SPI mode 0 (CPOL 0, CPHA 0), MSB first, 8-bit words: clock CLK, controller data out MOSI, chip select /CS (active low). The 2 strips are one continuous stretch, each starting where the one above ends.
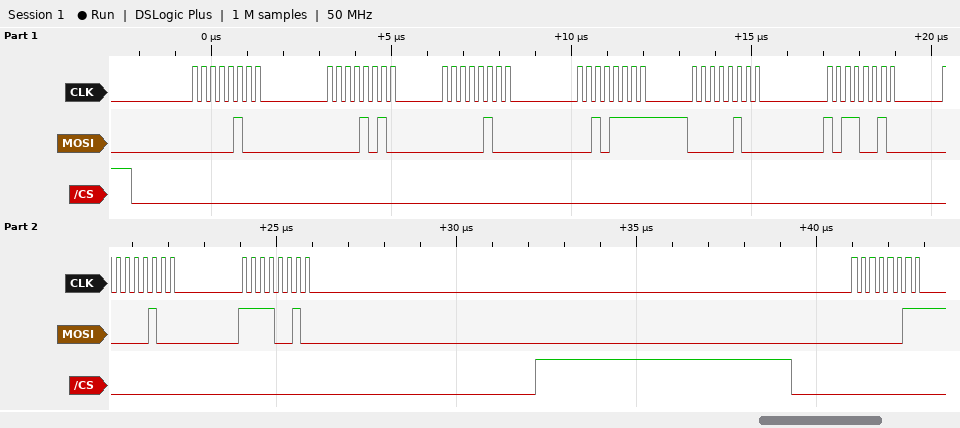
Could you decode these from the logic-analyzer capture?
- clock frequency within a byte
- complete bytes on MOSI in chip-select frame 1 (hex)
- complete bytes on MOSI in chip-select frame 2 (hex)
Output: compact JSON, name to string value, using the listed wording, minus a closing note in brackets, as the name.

{"clock frequency within a byte": "4 MHz", "complete bytes on MOSI in chip-select frame 1": "04 0A 04 2F 04 B2 04 F2", "complete bytes on MOSI in chip-select frame 2": "03"}
